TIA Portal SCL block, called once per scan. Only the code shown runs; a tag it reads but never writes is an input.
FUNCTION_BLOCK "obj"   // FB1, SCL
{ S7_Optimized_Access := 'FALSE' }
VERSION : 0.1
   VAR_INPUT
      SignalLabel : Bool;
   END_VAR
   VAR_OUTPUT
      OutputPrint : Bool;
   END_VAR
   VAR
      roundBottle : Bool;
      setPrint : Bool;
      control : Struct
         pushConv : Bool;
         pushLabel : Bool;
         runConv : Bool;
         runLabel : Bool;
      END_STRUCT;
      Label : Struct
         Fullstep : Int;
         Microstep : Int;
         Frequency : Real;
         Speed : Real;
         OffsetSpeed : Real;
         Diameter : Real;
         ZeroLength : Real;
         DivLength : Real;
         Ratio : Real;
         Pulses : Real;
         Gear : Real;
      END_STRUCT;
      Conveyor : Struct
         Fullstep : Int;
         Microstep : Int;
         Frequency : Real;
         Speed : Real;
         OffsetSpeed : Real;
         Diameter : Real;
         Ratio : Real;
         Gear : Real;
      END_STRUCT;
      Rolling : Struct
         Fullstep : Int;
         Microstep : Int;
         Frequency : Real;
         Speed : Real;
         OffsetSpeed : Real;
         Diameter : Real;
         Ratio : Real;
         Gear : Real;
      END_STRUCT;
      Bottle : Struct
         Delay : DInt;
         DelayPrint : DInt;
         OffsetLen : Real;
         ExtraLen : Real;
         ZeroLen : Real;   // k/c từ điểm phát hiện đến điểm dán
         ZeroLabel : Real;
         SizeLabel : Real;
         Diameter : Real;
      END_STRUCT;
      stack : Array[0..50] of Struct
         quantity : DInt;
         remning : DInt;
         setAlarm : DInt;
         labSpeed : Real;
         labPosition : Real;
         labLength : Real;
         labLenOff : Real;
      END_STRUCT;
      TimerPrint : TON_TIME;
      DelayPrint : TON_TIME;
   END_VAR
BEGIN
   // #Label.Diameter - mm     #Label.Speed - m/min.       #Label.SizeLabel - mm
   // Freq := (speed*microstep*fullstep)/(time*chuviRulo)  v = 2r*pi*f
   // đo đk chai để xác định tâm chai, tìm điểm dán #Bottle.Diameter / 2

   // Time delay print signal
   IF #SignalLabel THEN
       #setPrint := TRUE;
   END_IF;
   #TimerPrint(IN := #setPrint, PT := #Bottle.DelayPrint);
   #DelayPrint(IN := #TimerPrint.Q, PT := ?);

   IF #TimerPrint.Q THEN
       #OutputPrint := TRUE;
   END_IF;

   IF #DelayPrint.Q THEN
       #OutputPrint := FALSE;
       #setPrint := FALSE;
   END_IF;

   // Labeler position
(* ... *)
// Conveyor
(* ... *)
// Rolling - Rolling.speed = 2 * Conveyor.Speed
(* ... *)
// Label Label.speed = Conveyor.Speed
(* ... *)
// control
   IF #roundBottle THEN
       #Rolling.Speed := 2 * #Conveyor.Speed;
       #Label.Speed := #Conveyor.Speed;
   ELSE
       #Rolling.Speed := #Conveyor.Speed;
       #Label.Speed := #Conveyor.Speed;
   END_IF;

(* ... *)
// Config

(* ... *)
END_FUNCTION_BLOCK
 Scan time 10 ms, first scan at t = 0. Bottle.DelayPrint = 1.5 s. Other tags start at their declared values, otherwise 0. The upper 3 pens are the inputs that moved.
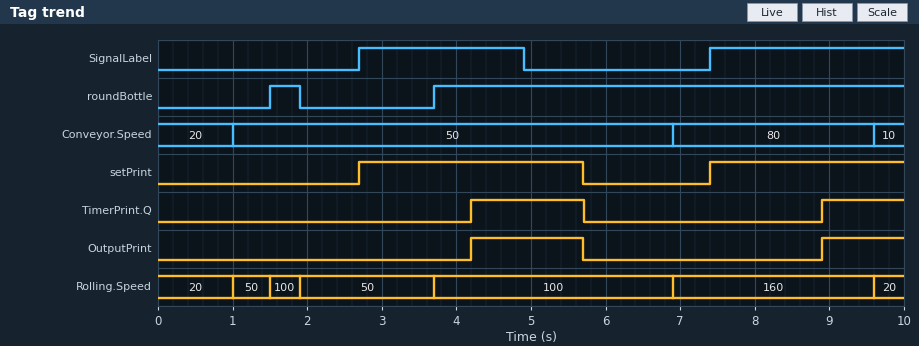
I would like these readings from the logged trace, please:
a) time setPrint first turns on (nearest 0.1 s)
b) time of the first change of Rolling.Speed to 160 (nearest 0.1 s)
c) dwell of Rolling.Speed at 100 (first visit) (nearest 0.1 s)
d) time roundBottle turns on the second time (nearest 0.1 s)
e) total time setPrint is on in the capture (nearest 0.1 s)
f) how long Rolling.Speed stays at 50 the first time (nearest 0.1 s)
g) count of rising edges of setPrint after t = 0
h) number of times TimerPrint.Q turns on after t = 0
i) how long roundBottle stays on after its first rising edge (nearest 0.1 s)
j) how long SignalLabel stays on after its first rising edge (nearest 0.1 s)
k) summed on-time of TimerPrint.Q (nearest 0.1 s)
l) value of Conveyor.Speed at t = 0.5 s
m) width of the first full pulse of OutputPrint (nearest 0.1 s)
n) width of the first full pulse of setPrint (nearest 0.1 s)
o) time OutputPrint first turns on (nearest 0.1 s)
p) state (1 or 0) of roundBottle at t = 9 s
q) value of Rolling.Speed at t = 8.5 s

2.7 s
6.9 s
0.4 s
3.7 s
5.6 s
0.5 s
2
2
0.4 s
2.2 s
2.6 s
20
1.5 s
3.0 s
4.2 s
1
160
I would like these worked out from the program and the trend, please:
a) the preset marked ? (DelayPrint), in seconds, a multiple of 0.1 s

1.5 s
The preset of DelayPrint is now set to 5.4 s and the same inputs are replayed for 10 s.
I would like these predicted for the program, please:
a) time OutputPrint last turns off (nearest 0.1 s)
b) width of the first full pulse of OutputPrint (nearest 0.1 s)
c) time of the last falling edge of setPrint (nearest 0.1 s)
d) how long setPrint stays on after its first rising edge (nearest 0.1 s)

9.6 s
5.4 s
9.6 s
6.9 s
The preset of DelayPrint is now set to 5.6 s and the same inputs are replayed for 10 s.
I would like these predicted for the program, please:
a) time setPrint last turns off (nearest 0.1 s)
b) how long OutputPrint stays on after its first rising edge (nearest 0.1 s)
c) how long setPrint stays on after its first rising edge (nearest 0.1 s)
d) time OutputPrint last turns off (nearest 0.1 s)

9.8 s
5.6 s
7.1 s
9.8 s
